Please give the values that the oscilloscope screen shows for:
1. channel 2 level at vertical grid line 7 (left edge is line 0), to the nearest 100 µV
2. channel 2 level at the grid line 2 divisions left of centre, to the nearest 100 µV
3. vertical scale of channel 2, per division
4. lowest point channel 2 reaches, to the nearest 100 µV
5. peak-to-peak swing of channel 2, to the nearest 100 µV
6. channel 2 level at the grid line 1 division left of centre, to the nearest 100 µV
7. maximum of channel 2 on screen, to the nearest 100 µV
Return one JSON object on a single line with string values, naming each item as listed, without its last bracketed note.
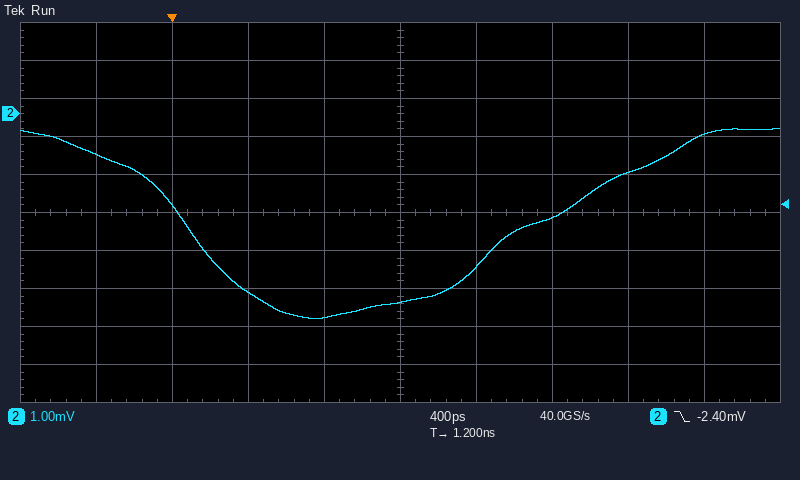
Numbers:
{"channel 2 level at vertical grid line 7 (left edge is line 0), to the nearest 100 µV": "-2.7 mV", "channel 2 level at the grid line 2 divisions left of centre, to the nearest 100 µV": "-4.7 mV", "vertical scale of channel 2, per division": "1 mV", "lowest point channel 2 reaches, to the nearest 100 µV": "-5.4 mV", "peak-to-peak swing of channel 2, to the nearest 100 µV": "5.0 mV", "channel 2 level at the grid line 1 division left of centre, to the nearest 100 µV": "-5.4 mV", "maximum of channel 2 on screen, to the nearest 100 µV": "-400 µV"}
